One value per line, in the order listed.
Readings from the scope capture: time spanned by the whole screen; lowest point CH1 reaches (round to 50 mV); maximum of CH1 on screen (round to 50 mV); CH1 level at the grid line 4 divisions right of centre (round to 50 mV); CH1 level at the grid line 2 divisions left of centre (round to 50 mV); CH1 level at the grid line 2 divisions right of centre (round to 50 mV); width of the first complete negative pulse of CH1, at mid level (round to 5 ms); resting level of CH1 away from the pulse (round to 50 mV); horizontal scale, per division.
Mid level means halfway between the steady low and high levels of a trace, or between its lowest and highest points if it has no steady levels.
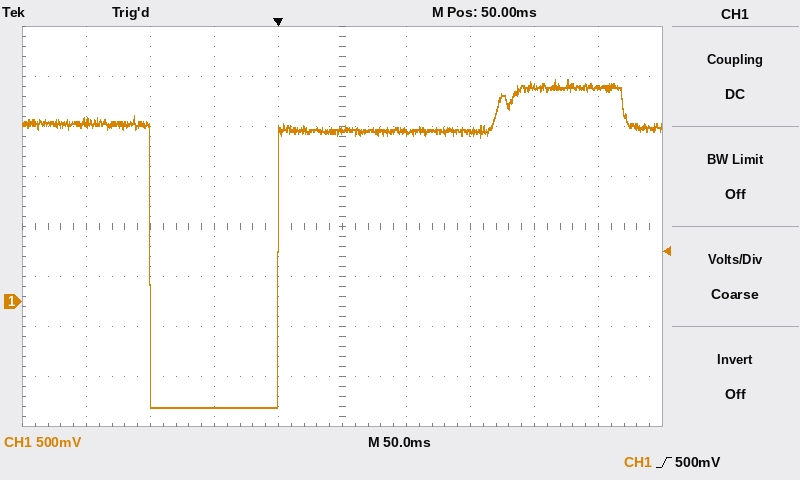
500 ms
-1.05 V
2.20 V
2.15 V
-1.05 V
1.70 V
100 ms
1.70 V
50 ms
